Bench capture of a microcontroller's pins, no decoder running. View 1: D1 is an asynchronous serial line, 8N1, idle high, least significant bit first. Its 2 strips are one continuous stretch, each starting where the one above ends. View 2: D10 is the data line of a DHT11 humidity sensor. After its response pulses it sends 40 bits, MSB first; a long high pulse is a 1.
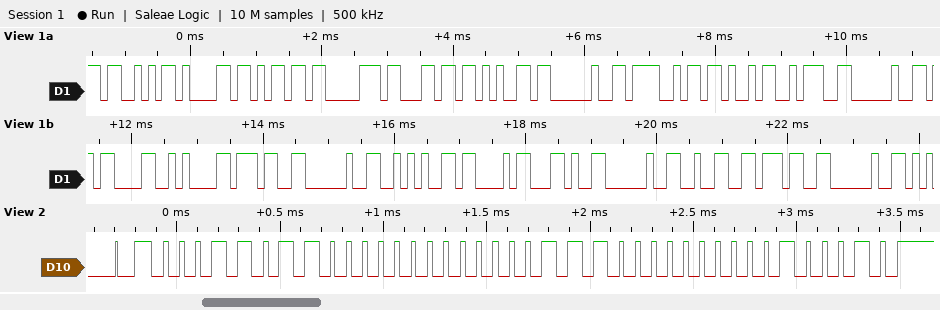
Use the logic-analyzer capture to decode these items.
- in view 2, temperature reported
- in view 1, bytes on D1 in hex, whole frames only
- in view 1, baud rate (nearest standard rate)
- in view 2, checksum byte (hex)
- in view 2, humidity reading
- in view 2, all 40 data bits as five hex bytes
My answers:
7.0 °C
53 61 6D 70 6C 65 20 4F 4B 3A 20 0D 0A 37 20 2A 43 2C 20 32 37 20
9600 baud
0x22
27 %
1B 00 07 00 22
